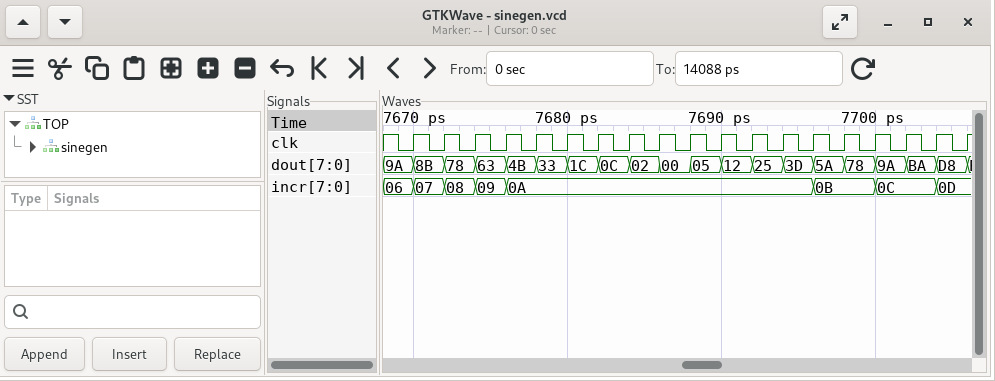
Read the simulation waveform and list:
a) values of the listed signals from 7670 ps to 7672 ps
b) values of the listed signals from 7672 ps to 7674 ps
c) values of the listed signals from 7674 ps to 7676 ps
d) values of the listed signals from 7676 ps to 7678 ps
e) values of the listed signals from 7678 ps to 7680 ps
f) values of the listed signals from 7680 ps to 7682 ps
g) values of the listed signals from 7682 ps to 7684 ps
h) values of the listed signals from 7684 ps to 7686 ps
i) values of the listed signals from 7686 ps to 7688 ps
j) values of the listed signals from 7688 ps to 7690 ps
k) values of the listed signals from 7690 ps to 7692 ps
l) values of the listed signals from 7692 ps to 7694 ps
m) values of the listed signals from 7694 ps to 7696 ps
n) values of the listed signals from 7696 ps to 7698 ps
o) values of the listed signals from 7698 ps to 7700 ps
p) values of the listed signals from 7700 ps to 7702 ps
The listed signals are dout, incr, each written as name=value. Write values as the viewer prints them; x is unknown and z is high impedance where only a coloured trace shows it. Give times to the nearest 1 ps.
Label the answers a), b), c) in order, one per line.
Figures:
a) dout=8B, incr=07
b) dout=78, incr=08
c) dout=63, incr=09
d) dout=4B, incr=0A
e) dout=33, incr=0A
f) dout=1C, incr=0A
g) dout=0C, incr=0A
h) dout=02, incr=0A
i) dout=00, incr=0A
j) dout=05, incr=0A
k) dout=12, incr=0A
l) dout=25, incr=0A
m) dout=3D, incr=0A
n) dout=5A, incr=0B
o) dout=78, incr=0B
p) dout=9A, incr=0C
